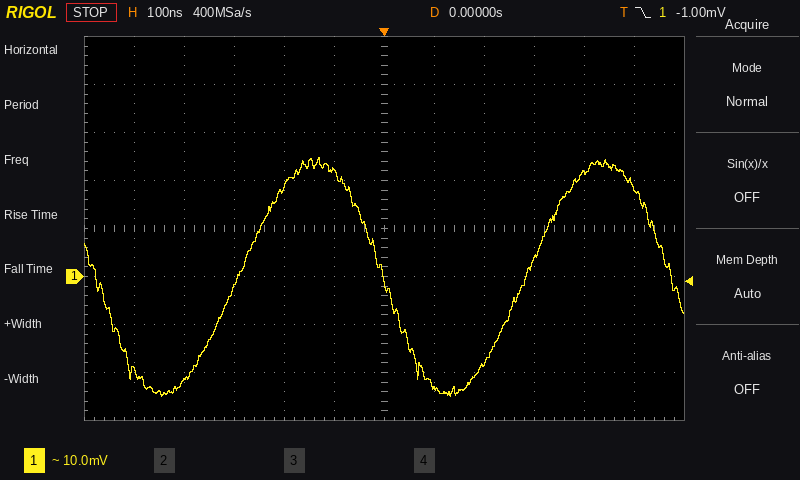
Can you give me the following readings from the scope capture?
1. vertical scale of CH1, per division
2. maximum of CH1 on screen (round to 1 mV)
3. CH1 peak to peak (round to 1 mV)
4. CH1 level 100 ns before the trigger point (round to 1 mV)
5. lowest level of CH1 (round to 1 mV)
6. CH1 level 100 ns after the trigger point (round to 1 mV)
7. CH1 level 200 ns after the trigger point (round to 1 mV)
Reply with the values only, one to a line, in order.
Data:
10 mV
25 mV
50 mV
22 mV
-25 mV
-23 mV
-18 mV
